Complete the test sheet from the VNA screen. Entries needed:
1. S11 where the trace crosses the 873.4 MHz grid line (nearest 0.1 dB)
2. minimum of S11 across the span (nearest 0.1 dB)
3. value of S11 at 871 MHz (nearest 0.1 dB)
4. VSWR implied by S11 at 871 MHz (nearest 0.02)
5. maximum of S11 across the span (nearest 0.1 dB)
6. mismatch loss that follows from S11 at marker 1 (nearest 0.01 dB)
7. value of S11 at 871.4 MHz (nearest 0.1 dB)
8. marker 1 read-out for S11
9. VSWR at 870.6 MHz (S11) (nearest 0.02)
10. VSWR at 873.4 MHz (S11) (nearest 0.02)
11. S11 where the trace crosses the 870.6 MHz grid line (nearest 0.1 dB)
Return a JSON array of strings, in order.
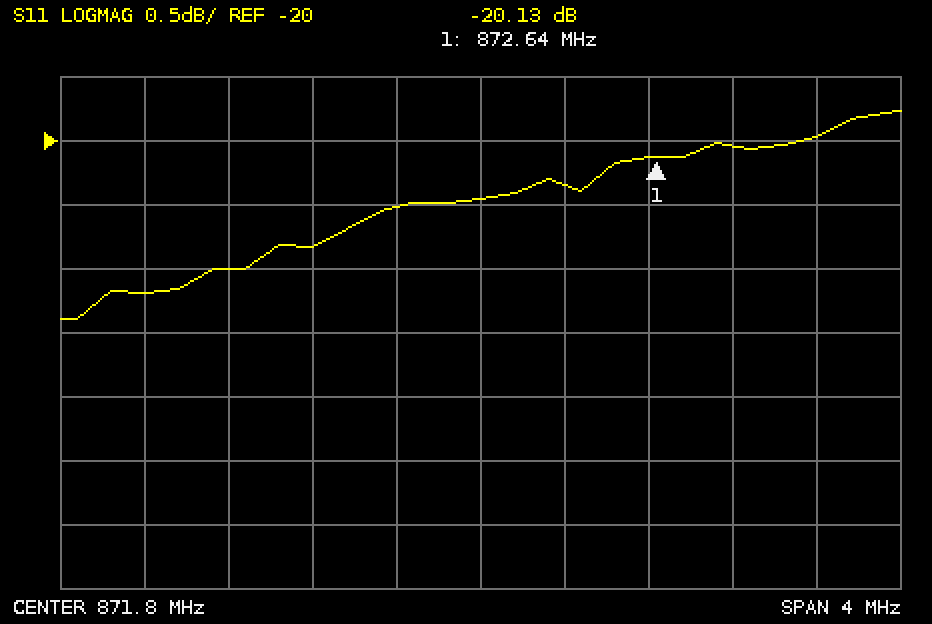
["-20.0 dB", "-21.4 dB", "-20.8 dB", "1.20", "-19.8 dB", "0.04 dB", "-20.5 dB", "-20.13 dB", "1.20", "1.22", "-21.0 dB"]
